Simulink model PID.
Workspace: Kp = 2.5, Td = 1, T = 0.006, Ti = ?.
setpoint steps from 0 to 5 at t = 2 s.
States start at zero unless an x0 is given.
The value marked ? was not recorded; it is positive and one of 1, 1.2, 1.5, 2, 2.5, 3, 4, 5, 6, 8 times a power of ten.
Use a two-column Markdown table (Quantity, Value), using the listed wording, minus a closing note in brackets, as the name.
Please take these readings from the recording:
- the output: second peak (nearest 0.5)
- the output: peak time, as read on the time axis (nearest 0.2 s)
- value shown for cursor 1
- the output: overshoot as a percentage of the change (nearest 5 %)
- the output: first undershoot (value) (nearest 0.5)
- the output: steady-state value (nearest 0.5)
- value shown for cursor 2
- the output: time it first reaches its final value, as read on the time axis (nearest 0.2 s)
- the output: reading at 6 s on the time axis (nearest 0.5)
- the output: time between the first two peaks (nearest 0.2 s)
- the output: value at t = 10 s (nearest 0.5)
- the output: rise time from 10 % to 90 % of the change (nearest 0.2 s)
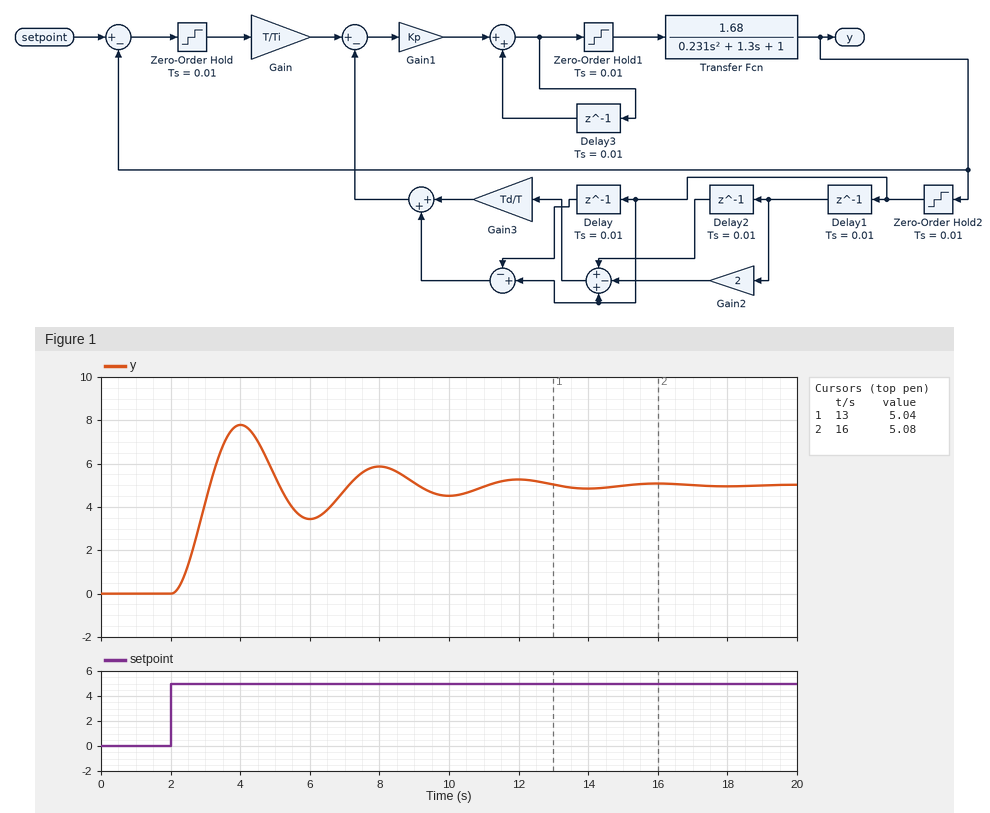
| Quantity | Value |
|---|---|
| the output: second peak | 6.0 |
| the output: peak time, as read on the time axis | 4.0 s |
| value shown for cursor 1 | 5.04 |
| the output: overshoot as a percentage of the change | 55 % |
| the output: first undershoot (value) | 3.5 |
| the output: steady-state value | 5.0 |
| value shown for cursor 2 | 5.08 |
| the output: time it first reaches its final value, as read on the time axis | 3.2 s |
| the output: reading at 6 s on the time axis | 3.5 |
| the output: time between the first two peaks | 4.0 s |
| the output: value at t = 10 s | 4.5 |
| the output: rise time from 10 % to 90 % of the change | 0.8 s |
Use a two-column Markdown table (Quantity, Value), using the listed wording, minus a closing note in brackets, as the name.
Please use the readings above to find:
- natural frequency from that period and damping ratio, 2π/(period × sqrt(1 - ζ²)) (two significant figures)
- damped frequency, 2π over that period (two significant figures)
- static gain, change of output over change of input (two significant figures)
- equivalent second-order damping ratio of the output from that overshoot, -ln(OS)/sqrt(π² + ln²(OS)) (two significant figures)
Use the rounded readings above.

| Quantity | Value |
|---|---|
| natural frequency from that period and damping ratio, 2π/(period × sqrt(1 - ζ²)) | 1.6 rad/s |
| damped frequency, 2π over that period | 1.6 rad/s |
| static gain, change of output over change of input | 1.0 |
| equivalent second-order damping ratio of the output from that overshoot, -ln(OS)/sqrt(π² + ln²(OS)) | 0.19 |
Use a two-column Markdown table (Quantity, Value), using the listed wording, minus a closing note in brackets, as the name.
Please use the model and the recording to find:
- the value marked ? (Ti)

| Quantity | Value |
|---|---|
| the value marked ? | 0.12 |
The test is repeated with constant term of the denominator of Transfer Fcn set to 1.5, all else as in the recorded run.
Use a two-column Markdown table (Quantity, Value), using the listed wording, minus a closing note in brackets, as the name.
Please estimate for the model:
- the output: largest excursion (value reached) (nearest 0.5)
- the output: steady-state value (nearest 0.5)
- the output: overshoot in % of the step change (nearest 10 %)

| Quantity | Value |
|---|---|
| the output: largest excursion (value reached) | 7.5 |
| the output: steady-state value | 5.0 |
| the output: overshoot in % of the step change | 50 % |
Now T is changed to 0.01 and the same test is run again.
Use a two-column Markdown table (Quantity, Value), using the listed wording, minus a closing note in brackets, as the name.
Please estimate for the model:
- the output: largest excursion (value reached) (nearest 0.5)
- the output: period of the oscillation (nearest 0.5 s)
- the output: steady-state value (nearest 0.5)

| Quantity | Value |
|---|---|
| the output: largest excursion (value reached) | 8.0 |
| the output: period of the oscillation | 2.5 s |
| the output: steady-state value | 5.0 |
